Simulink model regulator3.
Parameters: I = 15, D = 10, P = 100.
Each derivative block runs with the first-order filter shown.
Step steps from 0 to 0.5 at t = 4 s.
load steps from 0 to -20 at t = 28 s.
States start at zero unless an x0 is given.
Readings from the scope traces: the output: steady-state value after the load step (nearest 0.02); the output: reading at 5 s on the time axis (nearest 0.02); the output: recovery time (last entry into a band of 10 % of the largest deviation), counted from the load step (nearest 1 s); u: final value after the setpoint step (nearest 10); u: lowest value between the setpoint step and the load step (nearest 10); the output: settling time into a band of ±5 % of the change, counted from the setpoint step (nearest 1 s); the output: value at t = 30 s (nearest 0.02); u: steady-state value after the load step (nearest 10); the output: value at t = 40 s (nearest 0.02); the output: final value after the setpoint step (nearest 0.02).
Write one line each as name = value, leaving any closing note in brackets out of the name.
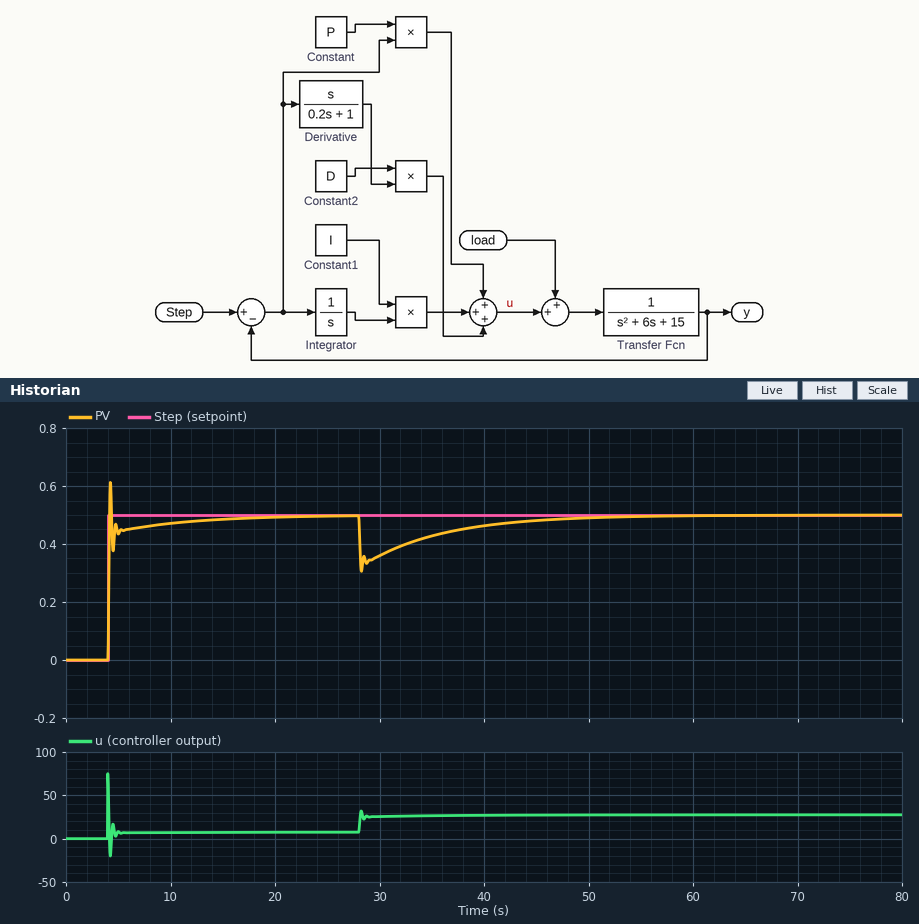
the output: steady-state value after the load step = 0.50
the output: reading at 5 s on the time axis = 0.44
the output: recovery time (last entry into a band of 10 % of the largest deviation), counted from the load step = 17 s
u: final value after the setpoint step = 10
u: lowest value between the setpoint step and the load step = -20
the output: settling time into a band of ±5 % of the change, counted from the setpoint step = 7 s
the output: value at t = 30 s = 0.36
u: steady-state value after the load step = 30
the output: value at t = 40 s = 0.46
the output: final value after the setpoint step = 0.50
